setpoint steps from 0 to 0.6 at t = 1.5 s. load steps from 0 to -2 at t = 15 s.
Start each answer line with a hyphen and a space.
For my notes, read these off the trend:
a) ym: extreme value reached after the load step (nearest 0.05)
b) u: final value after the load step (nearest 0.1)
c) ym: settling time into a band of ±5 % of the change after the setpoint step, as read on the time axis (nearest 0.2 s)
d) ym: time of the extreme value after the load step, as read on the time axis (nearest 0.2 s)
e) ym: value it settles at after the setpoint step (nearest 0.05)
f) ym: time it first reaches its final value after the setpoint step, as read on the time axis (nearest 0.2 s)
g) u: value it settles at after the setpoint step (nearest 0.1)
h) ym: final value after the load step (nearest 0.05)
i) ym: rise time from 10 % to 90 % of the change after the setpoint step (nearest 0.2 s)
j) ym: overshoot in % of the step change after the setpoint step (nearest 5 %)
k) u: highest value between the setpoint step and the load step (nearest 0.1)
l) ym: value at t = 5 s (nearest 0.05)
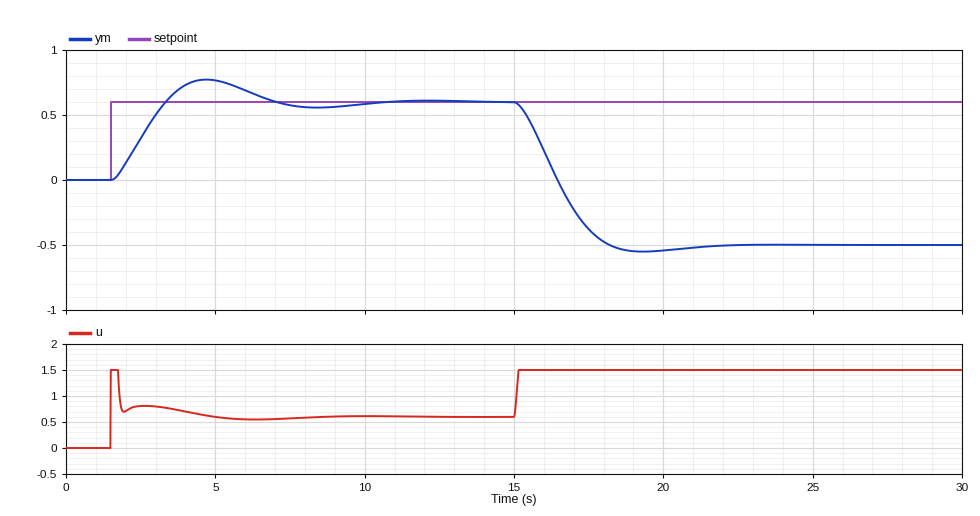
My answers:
- -0.55
- 1.5
- 9.4 s
- 19.4 s
- 0.60
- 3.4 s
- 0.6
- -0.50
- 1.4 s
- 30 %
- 1.5
- 0.75
